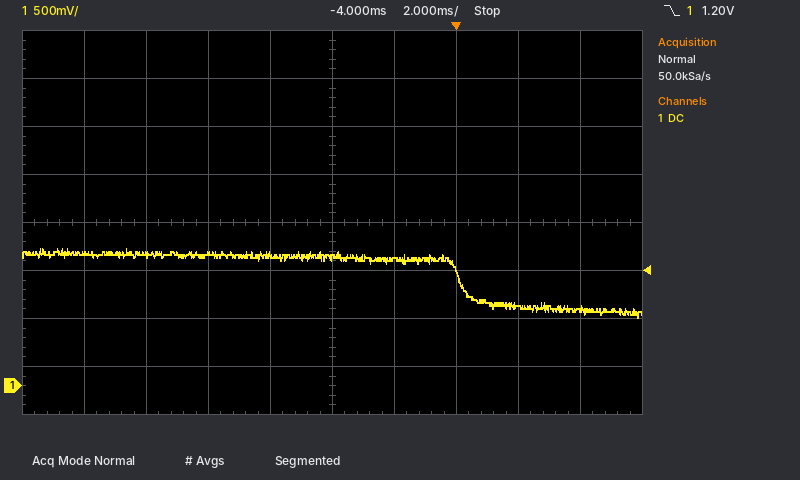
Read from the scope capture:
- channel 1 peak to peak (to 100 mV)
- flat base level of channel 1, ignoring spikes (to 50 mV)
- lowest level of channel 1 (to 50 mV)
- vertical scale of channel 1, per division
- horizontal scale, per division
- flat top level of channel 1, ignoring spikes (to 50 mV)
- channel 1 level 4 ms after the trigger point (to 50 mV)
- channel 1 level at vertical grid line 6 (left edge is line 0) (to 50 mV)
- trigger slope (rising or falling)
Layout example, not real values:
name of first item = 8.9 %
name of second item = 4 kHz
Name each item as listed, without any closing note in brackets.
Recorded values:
channel 1 peak to peak = 700 mV
flat base level of channel 1, ignoring spikes = 800 mV
lowest level of channel 1 = 700 mV
vertical scale of channel 1, per division = 500 mV
horizontal scale, per division = 2 ms
flat top level of channel 1, ignoring spikes = 1.35 V
channel 1 level 4 ms after the trigger point = 800 mV
channel 1 level at vertical grid line 6 (left edge is line 0) = 1.30 V
trigger slope = falling
